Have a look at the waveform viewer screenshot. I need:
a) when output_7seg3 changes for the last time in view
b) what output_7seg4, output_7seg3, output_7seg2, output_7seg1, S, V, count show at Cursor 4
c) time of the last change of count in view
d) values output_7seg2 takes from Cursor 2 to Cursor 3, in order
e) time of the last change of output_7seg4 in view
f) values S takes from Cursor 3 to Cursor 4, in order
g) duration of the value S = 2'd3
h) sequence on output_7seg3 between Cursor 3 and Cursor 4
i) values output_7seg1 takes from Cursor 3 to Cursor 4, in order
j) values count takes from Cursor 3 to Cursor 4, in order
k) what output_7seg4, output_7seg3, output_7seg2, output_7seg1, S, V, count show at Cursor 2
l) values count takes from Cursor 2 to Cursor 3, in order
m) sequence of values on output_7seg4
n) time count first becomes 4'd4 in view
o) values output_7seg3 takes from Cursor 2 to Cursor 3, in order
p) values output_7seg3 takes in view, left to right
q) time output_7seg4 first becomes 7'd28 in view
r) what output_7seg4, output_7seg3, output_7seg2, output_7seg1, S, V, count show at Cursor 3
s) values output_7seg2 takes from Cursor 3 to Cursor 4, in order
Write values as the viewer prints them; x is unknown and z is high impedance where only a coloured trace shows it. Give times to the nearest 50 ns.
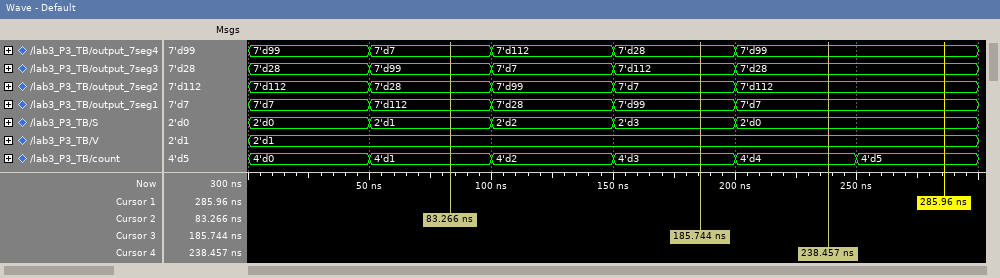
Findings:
200 ns
output_7seg4=7'd99, output_7seg3=7'd28, output_7seg2=7'd112, output_7seg1=7'd7, S=2'd0, V=2'd1, count=4'd4
250 ns
7'd28, 7'd99, 7'd7
200 ns
2'd3, 2'd0
50 ns
7'd112, 7'd28
7'd99, 7'd7
4'd3, 4'd4
output_7seg4=7'd7, output_7seg3=7'd99, output_7seg2=7'd28, output_7seg1=7'd112, S=2'd1, V=2'd1, count=4'd1
4'd1, 4'd2, 4'd3
7'd99, 7'd7, 7'd112, 7'd28, 7'd99
200 ns
7'd99, 7'd7, 7'd112
7'd28, 7'd99, 7'd7, 7'd112, 7'd28
150 ns
output_7seg4=7'd28, output_7seg3=7'd112, output_7seg2=7'd7, output_7seg1=7'd99, S=2'd3, V=2'd1, count=4'd3
7'd7, 7'd112
